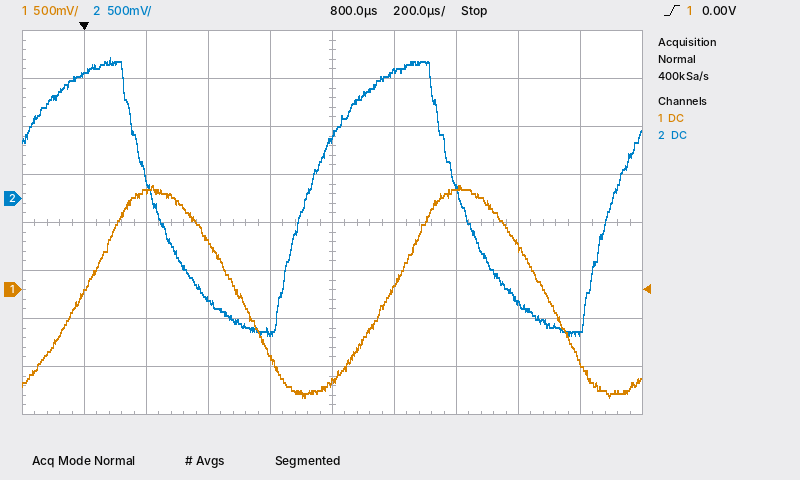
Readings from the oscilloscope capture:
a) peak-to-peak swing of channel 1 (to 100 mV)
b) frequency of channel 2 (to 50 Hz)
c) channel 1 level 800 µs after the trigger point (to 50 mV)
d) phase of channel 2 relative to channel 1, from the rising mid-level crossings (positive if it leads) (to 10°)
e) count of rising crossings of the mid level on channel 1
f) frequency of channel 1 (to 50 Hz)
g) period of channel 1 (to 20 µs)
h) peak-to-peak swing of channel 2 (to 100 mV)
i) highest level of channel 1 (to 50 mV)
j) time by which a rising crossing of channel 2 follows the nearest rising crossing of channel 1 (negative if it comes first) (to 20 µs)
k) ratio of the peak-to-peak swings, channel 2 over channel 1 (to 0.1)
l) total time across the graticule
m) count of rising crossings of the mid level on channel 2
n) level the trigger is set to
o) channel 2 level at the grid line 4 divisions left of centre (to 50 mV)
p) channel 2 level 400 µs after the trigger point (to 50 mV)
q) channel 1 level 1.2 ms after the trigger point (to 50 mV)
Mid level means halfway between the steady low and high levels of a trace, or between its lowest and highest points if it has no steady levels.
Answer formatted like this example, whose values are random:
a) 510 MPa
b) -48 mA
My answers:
a) 2.20 V
b) 1.00 kHz
c) -950 mV
d) +100°
e) 2
f) 1.00 kHz
g) 1.00 ms
h) 2.90 V
i) 1.10 V
j) -280 µs
k) 1.3
l) 2 ms
m) 2
n) 0.00 V
o) 1.30 V
p) -1.05 V
q) 1.05 V
